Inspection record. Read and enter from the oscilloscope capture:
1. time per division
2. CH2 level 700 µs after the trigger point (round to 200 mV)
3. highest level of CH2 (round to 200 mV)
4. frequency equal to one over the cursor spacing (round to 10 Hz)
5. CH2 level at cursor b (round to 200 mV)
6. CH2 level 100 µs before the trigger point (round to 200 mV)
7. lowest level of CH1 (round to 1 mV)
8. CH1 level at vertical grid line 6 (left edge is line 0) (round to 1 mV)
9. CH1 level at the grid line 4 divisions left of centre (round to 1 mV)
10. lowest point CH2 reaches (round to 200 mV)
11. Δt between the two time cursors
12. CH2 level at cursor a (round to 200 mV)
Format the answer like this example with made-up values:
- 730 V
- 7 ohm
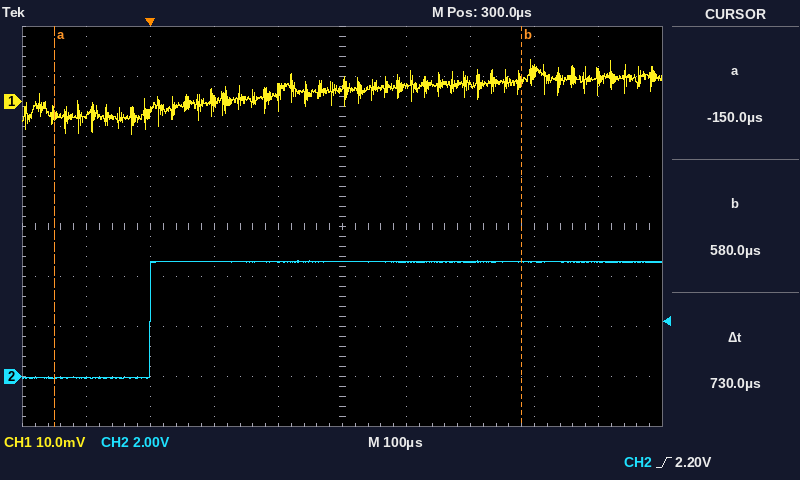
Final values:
- 100 µs
- 4.6 V
- 4.6 V
- 1.37 kHz
- 4.6 V
- 0.0 V
- -7 mV
- 3 mV
- -3 mV
- 0.0 V
- 730 µs
- 0.0 V
